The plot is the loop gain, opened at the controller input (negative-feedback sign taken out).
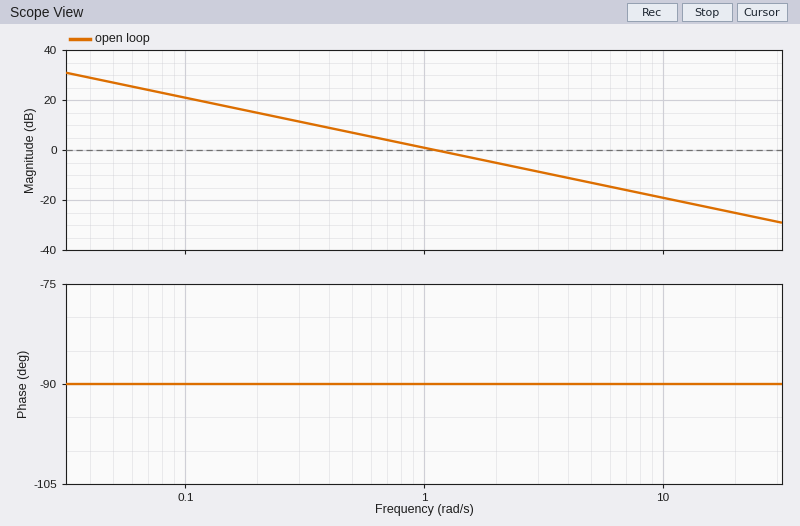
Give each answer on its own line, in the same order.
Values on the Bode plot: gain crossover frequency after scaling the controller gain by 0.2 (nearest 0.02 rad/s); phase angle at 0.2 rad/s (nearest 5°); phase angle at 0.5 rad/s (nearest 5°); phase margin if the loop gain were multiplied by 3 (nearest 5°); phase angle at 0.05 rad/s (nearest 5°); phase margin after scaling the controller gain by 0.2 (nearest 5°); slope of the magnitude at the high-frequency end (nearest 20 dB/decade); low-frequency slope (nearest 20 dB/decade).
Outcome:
0.22 rad/s
-90°
-90°
90°
-90°
90°
-20 dB/decade
-20 dB/decade
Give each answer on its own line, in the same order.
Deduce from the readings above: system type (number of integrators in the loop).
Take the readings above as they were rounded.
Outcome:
1
